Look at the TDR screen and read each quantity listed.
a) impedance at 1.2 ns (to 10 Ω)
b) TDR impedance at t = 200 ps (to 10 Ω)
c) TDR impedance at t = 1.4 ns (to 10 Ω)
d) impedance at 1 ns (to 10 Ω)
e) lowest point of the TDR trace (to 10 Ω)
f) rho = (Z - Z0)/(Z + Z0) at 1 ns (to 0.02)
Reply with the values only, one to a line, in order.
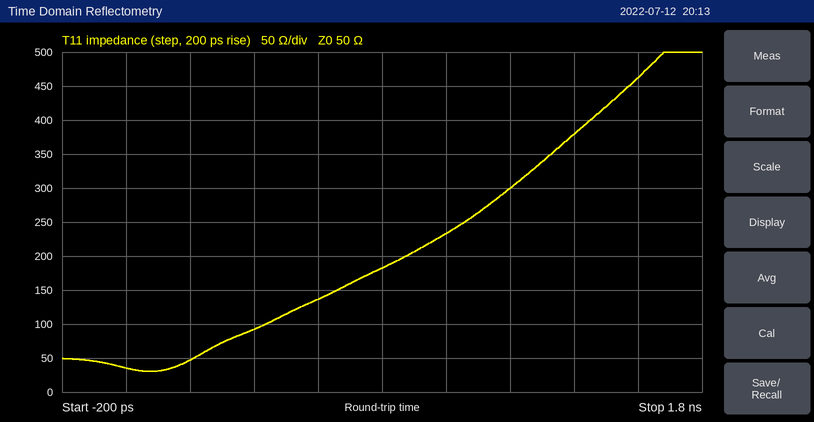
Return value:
300 Ω
50 Ω
380 Ω
230 Ω
30 Ω
+0.64
